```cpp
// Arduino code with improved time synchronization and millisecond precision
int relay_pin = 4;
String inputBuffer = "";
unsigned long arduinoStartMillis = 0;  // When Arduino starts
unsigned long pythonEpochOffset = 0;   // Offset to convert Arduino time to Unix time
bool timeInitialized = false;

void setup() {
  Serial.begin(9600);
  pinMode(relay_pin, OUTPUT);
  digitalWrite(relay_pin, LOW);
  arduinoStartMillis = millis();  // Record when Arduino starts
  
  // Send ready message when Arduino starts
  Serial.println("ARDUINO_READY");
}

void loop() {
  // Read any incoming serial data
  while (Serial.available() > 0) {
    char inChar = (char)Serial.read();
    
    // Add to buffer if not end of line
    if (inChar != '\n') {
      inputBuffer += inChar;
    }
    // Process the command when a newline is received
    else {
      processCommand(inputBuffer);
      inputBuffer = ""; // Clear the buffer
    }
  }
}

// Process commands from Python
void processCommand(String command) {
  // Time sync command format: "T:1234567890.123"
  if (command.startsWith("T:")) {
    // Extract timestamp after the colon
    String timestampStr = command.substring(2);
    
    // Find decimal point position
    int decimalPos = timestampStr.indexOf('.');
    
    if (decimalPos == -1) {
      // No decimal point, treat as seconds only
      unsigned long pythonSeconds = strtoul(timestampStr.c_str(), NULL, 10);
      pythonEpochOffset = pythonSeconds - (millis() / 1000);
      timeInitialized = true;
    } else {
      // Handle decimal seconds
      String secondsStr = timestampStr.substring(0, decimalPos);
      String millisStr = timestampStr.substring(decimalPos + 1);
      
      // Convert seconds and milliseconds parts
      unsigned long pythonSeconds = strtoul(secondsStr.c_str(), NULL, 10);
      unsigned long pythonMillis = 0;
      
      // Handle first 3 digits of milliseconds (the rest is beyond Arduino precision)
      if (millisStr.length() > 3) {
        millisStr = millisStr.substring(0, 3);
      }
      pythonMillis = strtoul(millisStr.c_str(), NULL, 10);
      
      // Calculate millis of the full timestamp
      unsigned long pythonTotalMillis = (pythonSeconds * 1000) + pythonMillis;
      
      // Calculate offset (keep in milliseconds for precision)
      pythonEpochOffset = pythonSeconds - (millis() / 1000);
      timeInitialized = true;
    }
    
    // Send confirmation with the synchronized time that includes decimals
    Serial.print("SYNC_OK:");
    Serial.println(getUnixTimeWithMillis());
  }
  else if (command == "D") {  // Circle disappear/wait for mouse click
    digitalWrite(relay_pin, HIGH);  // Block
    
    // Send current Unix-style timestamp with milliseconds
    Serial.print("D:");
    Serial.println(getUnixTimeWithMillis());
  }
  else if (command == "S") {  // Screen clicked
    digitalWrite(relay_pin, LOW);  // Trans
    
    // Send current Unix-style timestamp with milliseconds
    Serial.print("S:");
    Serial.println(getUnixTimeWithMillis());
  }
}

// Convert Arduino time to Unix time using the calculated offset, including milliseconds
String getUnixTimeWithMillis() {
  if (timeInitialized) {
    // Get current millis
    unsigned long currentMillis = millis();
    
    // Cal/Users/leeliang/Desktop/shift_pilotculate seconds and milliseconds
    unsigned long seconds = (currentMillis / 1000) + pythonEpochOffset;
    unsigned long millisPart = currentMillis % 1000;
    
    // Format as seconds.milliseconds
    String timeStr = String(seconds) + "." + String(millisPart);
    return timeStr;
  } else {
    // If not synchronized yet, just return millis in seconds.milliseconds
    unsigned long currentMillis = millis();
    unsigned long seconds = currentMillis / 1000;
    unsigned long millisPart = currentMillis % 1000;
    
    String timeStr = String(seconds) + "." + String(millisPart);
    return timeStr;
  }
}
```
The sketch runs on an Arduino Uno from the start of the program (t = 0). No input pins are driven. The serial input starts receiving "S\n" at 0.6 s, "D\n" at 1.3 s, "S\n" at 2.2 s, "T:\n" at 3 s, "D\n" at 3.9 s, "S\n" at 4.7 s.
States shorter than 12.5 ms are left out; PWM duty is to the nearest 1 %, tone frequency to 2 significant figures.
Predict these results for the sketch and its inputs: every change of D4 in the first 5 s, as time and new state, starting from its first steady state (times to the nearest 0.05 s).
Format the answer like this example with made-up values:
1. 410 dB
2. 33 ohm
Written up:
1. 0 s low; 1.3 s high; 2.2 s low; 3.9 s high; 4.7 s low
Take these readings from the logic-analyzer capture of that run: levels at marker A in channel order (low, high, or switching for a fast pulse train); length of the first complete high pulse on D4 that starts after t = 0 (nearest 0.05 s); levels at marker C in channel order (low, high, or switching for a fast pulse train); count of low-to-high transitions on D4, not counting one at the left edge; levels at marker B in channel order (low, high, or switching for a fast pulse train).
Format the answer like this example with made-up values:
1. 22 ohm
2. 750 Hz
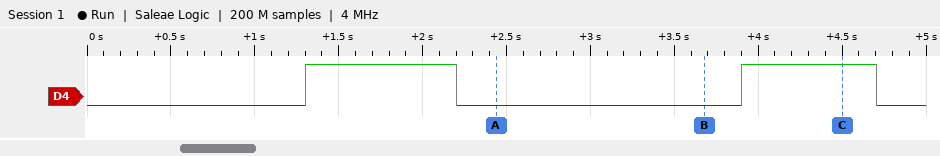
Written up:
1. D4 low
2. 0.90 s
3. D4 high
4. 2
5. D4 low
